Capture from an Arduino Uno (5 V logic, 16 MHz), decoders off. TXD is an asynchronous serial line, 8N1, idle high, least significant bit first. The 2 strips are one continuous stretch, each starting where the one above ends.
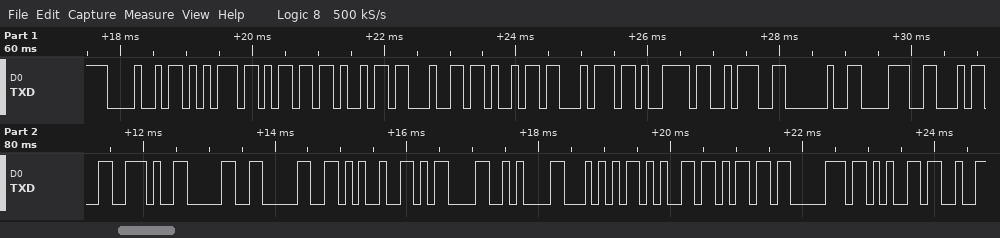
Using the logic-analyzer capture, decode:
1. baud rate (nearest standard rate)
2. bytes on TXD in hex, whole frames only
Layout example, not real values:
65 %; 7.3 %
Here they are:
9600 baud; 48 75 6D 69 64 69 74 79 3A 20 38 34 2E 30 30 25 0D 0A 54 65 6D 70 65
